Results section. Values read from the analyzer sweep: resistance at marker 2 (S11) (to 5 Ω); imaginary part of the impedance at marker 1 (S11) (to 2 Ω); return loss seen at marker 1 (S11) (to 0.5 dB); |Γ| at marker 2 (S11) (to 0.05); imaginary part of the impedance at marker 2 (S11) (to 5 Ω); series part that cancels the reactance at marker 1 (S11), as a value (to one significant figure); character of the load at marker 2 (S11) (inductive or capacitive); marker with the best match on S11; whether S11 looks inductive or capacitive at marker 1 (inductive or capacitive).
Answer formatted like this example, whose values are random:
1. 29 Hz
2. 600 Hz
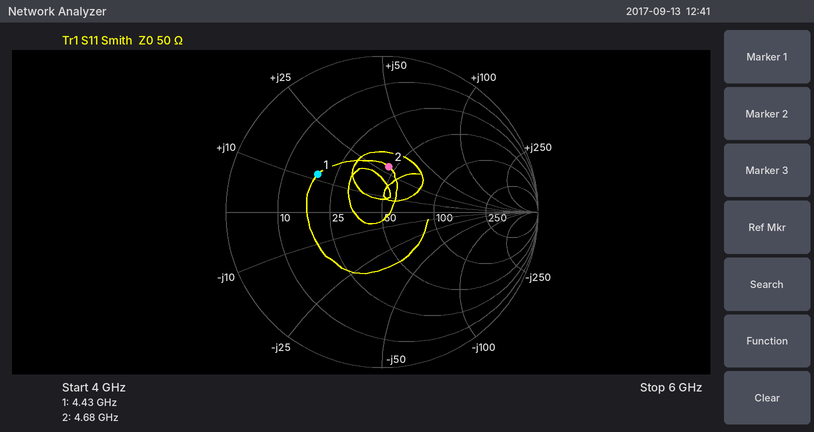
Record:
1. 45 Ω
2. +12 Ω
3. 6.5 dB
4. 0.30
5. +30 Ω
6. 3 pF
7. inductive
8. marker 2
9. inductive
